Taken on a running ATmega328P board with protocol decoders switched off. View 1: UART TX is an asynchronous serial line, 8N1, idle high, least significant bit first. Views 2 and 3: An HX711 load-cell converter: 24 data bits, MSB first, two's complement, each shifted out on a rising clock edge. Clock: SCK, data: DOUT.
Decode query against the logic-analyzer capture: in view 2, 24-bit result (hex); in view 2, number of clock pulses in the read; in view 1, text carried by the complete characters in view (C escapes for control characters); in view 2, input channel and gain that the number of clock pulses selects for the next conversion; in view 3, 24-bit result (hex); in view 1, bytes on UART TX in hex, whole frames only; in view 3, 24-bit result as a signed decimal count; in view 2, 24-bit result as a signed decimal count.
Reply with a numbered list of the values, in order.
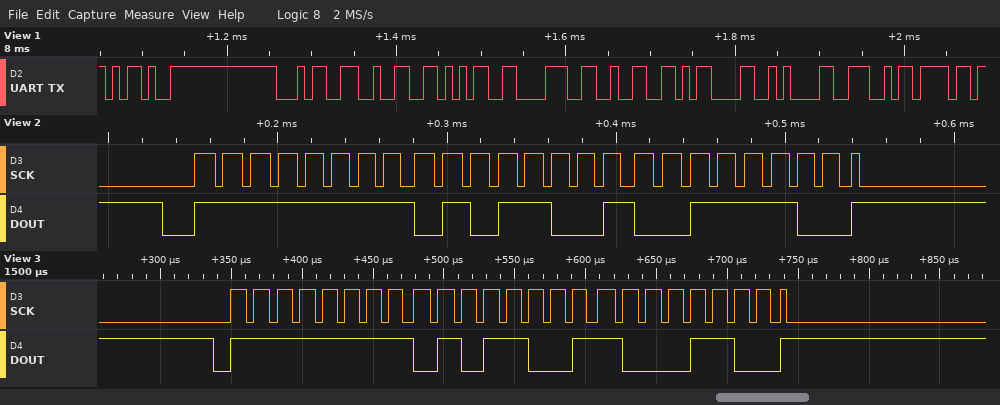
1. 0xFF593C
2. 25
3. "-42582\r\nNo"
4. channel A, gain 128
5. 0xFF598C
6. 2D 34 32 35 38 32 0D 0A 4E 6F
7. -42612
8. -42692
